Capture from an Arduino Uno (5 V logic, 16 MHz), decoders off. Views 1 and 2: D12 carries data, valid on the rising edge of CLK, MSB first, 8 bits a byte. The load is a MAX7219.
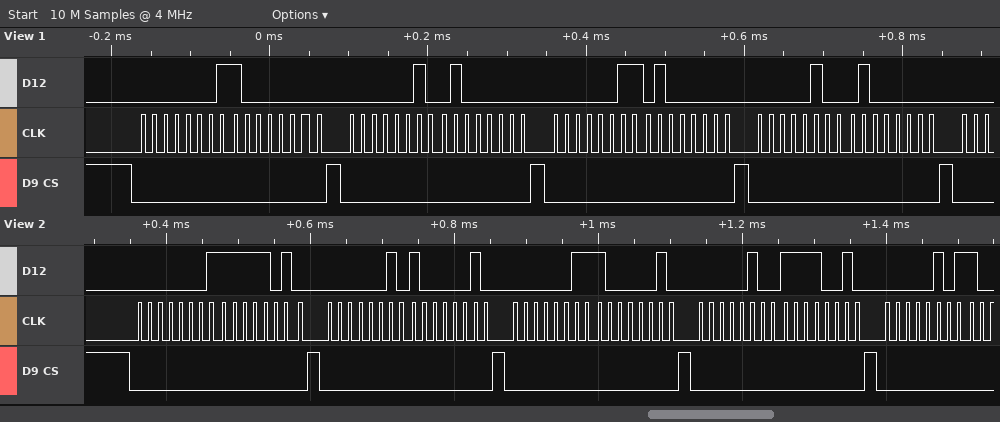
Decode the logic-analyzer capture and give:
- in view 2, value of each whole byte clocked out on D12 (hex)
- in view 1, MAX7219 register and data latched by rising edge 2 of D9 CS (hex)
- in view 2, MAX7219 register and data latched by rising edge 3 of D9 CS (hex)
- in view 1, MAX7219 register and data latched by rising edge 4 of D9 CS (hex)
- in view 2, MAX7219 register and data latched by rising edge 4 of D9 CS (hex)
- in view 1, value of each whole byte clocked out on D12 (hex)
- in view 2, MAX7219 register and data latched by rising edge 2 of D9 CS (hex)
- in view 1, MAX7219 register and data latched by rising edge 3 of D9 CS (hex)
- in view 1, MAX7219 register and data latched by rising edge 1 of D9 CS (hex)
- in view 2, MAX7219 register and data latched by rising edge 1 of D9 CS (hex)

01 FA 02 82 03 82 04 F2 05
register 0x2, data 0x40
register 0x3, data 0x82
register 0x4, data 0x40
register 0x4, data 0xF2
01 80 02 40 03 40 04 40
register 0x2, data 0x82
register 0x3, data 0x40
register 0x1, data 0x80
register 0x1, data 0xFA
